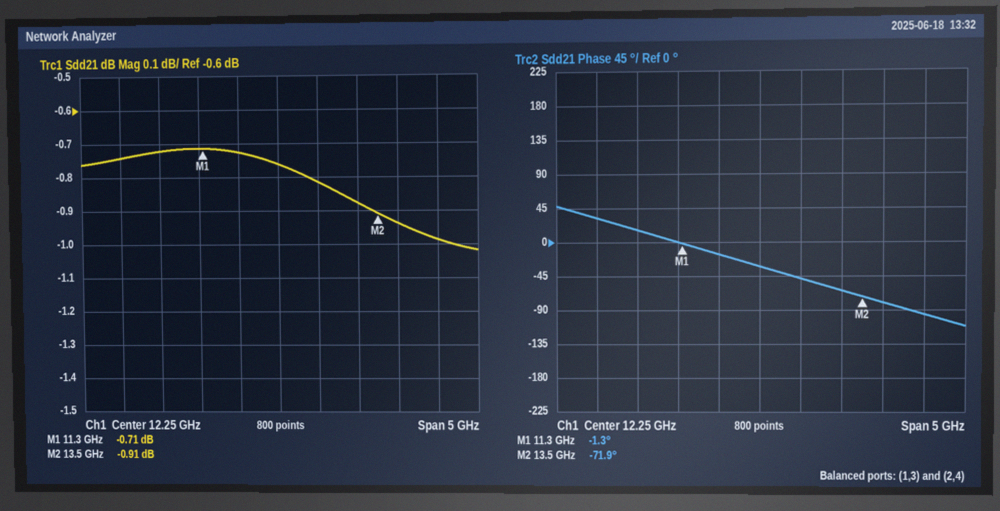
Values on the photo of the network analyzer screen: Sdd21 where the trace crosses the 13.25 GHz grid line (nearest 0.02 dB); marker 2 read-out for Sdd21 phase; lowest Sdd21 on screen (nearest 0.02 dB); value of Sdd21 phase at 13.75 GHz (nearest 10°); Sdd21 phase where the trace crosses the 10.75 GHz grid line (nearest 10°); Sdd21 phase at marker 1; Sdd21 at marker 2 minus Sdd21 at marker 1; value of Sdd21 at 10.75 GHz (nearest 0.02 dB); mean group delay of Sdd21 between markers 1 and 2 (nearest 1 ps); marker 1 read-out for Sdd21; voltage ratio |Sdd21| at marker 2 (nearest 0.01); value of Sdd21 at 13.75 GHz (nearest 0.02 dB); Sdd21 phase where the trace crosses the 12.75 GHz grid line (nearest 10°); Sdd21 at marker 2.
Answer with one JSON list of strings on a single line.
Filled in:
["-0.88 dB", "-71.9°", "-1.02 dB", "-80°", "20°", "-1.3°", "-0.20 dB", "-0.72 dB", "89 ps", "-0.71 dB", "0.90", "-0.94 dB", "-50°", "-0.91 dB"]
